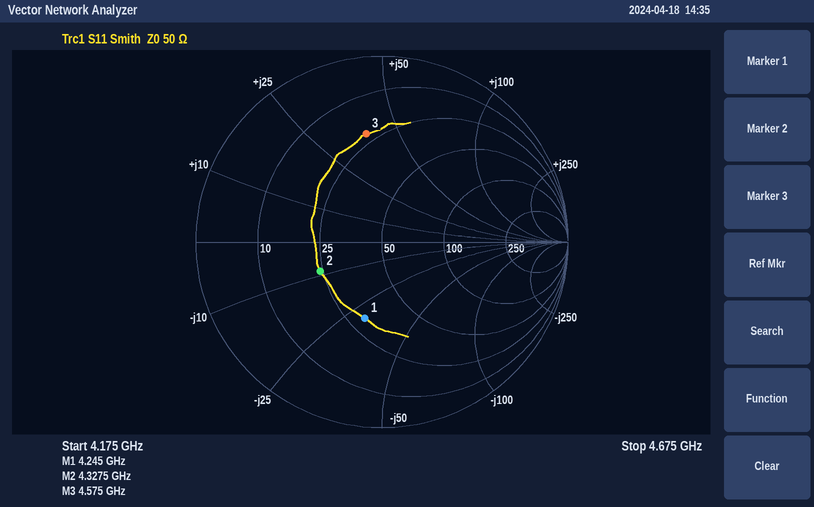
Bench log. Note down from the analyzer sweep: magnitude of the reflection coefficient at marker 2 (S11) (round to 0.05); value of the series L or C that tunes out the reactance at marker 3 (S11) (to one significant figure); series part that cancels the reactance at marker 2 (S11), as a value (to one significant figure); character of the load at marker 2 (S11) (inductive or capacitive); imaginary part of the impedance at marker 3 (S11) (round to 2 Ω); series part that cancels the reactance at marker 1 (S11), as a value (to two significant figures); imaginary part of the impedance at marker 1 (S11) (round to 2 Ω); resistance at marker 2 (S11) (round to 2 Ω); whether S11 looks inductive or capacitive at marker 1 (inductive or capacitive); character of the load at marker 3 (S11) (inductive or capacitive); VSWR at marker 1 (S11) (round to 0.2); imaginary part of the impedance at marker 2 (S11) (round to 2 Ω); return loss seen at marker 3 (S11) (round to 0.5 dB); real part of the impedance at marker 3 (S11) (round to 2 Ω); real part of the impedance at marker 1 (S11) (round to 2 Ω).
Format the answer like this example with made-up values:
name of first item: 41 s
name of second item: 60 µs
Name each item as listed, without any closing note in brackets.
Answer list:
magnitude of the reflection coefficient at marker 2 (S11): 0.35
value of the series L or C that tunes out the reactance at marker 3 (S11): 900 fF
series part that cancels the reactance at marker 2 (S11), as a value: 300 pH
character of the load at marker 2 (S11): capacitive
imaginary part of the impedance at marker 3 (S11): +38 Ω
series part that cancels the reactance at marker 1 (S11), as a value: 1.1 nH
imaginary part of the impedance at marker 1 (S11): -30 Ω
resistance at marker 2 (S11): 24 Ω
whether S11 looks inductive or capacitive at marker 1: capacitive
character of the load at marker 3 (S11): inductive
VSWR at marker 1 (S11): 2.4
imaginary part of the impedance at marker 2 (S11): -8 Ω
return loss seen at marker 3 (S11): 4.5 dB
real part of the impedance at marker 3 (S11): 22 Ω
real part of the impedance at marker 1 (S11): 30 Ω
